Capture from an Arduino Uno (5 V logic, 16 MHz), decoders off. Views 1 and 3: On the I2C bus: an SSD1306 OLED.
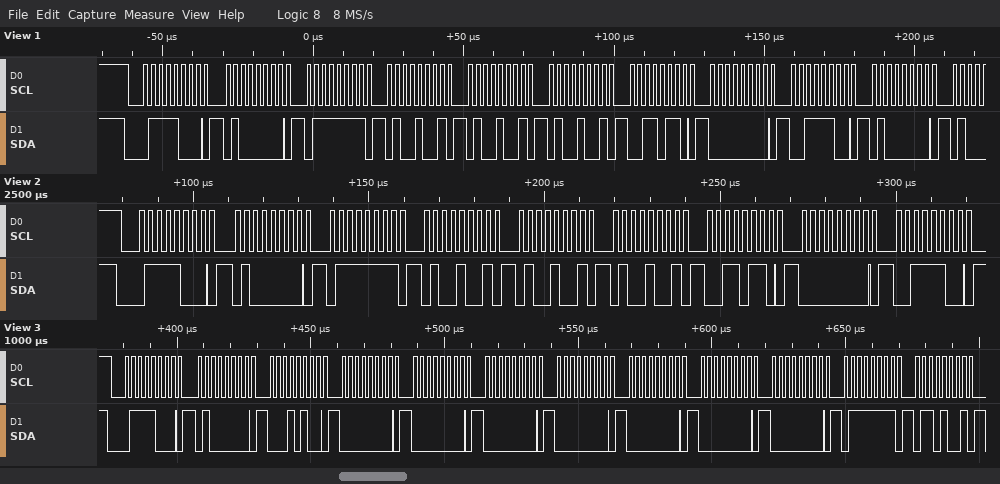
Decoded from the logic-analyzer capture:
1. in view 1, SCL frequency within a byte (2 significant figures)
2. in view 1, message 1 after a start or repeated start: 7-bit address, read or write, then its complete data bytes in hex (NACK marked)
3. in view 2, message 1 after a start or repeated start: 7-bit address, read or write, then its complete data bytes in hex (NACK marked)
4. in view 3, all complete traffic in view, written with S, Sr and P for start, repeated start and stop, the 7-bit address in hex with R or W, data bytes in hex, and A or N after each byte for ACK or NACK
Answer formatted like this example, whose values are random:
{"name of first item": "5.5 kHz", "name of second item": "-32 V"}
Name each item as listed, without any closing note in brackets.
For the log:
{"in view 1, SCL frequency within a byte": "400 kHz", "in view 1, message 1 after a start or repeated start: 7-bit address, read or write, then its complete data bytes in hex": "0x3C write: 40 7F 49 49 49 36 00 3C 40", "in view 2, message 1 after a start or repeated start: 7-bit address, read or write, then its complete data bytes in hex": "0x3C write: 40 7F 49 49 49 36 00 3C", "in view 3, all complete traffic in view, written with S, Sr and P for start, repeated start and stop, the 7-bit address in hex with R or W, data bytes in hex, and A or N after each byte for ACK or NACK": "S 3CW A 40 A 14 A 00 A 00 A 00 A 00 A 00 A 00 A 00 A 7F A 69 A"}
